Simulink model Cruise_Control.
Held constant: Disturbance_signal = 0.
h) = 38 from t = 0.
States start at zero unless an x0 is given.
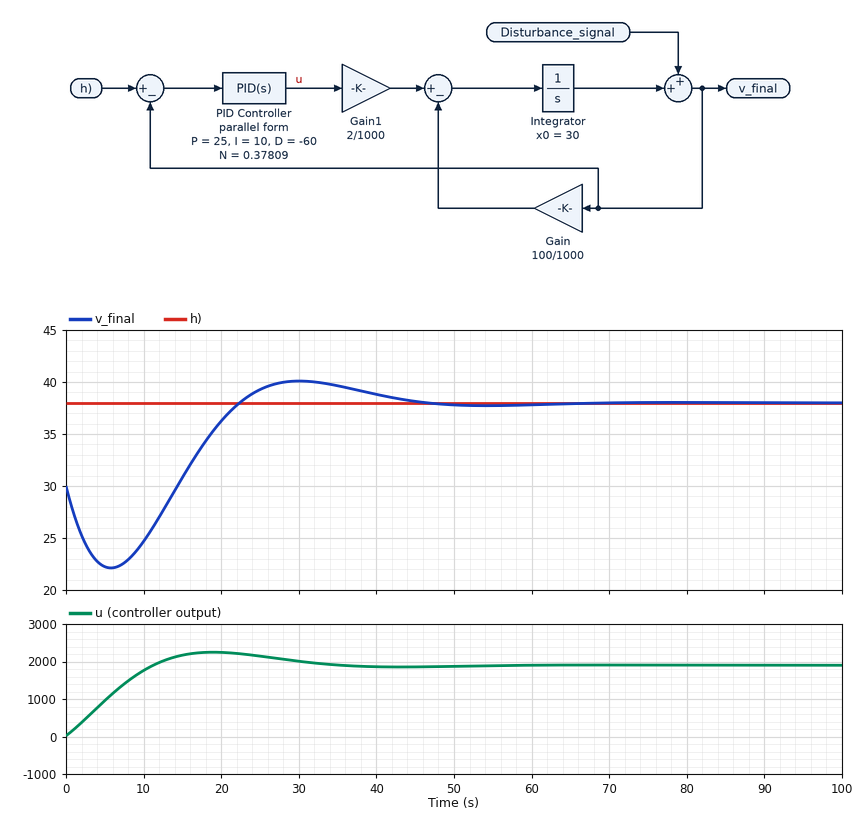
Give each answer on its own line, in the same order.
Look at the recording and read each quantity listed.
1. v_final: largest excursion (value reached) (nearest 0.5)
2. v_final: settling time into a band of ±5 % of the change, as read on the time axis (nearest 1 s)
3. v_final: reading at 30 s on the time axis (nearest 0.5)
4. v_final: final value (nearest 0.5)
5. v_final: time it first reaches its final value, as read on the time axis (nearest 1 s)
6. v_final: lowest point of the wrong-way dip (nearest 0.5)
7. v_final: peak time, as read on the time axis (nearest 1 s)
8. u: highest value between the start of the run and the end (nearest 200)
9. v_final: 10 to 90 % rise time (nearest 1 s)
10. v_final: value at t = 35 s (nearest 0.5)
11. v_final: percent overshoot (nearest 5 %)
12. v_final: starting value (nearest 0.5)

40.0
43 s
40.0
38.0
22 s
22.0
30 s
2200
6 s
39.5
25 %
30.0
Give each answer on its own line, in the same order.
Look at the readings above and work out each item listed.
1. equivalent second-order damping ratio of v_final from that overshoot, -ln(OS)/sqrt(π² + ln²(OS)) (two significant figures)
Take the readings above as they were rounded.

0.40
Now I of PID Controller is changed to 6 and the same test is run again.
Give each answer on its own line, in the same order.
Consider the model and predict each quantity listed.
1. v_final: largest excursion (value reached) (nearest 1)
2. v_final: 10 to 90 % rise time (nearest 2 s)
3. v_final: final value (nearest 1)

39
12 s
38
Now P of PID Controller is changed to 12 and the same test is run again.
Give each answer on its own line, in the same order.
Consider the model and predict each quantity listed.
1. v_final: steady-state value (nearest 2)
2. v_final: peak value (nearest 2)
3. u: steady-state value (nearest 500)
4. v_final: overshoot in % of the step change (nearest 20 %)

38
42
2000
40 %
